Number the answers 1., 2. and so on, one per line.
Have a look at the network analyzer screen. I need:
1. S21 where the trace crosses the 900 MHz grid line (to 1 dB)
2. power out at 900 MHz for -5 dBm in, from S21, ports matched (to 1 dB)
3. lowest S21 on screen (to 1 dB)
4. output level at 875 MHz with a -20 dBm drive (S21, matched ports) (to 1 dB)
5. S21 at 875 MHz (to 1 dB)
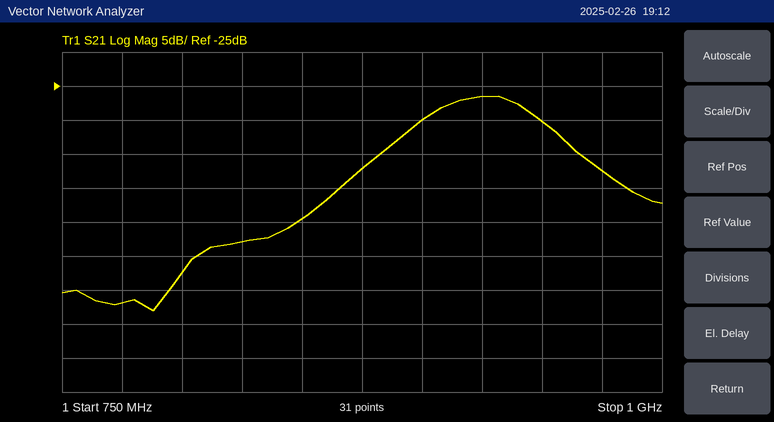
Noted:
1. -30 dB
2. -35 dBm
3. -58 dB
4. -57 dBm
5. -37 dB
